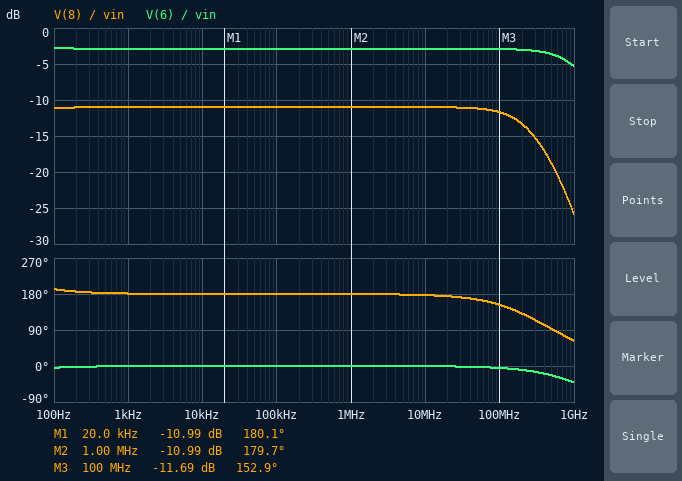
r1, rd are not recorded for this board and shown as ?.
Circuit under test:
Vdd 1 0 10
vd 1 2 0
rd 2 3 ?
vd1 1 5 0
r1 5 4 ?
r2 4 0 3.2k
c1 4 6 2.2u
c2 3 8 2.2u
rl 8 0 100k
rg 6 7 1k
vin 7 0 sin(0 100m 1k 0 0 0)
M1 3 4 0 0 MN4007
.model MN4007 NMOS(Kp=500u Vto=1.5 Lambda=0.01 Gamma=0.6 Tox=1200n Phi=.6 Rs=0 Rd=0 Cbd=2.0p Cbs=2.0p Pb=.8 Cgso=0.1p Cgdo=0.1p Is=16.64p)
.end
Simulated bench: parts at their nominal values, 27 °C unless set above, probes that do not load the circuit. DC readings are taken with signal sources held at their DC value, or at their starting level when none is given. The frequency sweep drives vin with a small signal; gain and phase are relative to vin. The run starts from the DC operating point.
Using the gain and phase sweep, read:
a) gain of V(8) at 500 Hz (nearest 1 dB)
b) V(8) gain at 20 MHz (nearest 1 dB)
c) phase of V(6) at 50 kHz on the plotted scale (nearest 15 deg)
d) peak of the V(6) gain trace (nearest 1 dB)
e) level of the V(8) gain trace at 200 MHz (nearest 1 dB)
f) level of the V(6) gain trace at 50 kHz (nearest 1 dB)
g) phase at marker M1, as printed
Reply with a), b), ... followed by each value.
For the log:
a) -11 dB
b) -11 dB
c) 0 deg
d) -3 dB
e) -13 dB
f) -3 dB
g) 180.1 deg
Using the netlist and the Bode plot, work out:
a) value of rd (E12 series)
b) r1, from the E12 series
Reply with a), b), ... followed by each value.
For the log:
a) 1.2 kΩ
b) 12 kΩ
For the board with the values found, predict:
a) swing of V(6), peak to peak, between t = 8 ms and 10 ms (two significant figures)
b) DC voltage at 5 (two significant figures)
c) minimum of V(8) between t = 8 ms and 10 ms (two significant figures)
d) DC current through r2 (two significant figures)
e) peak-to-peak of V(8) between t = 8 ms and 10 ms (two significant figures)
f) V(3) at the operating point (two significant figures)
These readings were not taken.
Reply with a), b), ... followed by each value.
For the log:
a) 140 mV
b) 10 V
c) -30 mV
d) 660 µA
e) 56 mV
f) 9.9 V
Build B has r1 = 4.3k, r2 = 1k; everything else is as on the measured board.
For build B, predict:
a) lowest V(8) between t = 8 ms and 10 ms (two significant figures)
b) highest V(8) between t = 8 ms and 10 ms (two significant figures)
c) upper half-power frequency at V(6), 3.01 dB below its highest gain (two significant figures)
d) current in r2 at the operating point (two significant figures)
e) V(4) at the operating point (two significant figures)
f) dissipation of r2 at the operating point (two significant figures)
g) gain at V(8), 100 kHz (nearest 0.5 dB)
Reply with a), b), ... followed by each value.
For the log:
a) -12 mV
b) 11 mV
c) 52 Hz
d) 1.9 mA
e) 1.9 V
f) 3.6 mW
g) -19.0 dB
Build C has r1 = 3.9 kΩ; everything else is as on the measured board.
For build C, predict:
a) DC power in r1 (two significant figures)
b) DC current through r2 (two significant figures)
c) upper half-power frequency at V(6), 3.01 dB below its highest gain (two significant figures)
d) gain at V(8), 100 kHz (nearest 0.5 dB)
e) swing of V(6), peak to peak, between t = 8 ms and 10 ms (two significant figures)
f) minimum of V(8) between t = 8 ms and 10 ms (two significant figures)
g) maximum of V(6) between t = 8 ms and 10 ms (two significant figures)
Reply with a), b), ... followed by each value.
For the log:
a) 7.7 mW
b) 1.4 mA
c) 61 Hz
d) 1.5 dB
e) 130 mV
f) -120 mV
g) 64 mV
